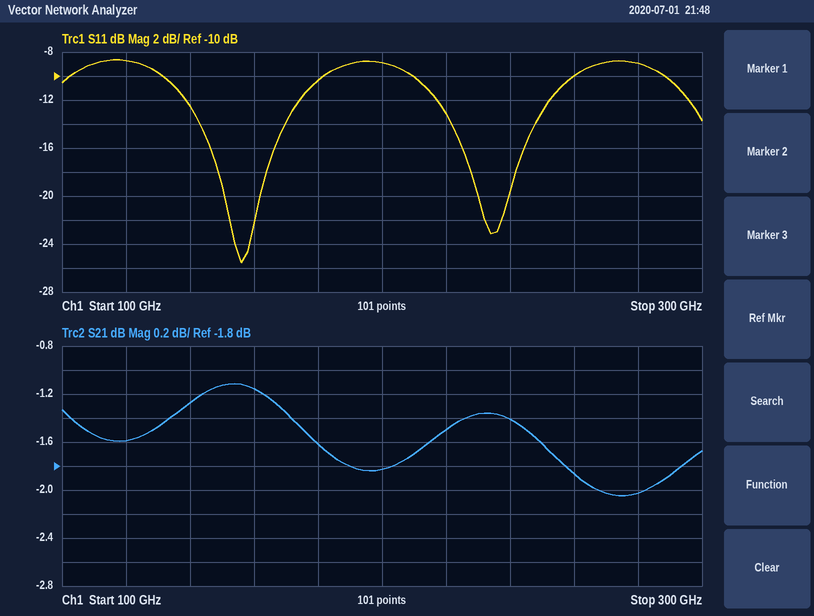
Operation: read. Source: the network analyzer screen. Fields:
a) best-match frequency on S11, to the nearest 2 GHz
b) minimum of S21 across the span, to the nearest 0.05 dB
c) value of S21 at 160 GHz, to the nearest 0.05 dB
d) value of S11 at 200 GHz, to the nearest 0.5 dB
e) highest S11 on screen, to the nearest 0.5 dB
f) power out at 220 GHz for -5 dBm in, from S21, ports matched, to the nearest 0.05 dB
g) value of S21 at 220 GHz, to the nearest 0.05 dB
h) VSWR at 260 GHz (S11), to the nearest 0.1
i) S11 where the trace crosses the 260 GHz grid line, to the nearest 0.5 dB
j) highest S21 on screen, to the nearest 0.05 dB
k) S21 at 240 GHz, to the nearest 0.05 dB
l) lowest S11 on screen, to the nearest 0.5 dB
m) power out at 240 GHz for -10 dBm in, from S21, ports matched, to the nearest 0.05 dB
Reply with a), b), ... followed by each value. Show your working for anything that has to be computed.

a) 156 GHz
b) -2.05 dB
c) -1.15 dB
d) -9.0 dB
e) -8.5 dB
f) -5 dBm + (-1.50 dB) = -6.50 dBm
g) -1.50 dB
h) |Γ| = 10^(-10/20) = 0.3162; VSWR = (1 + 0.3162)/(1 − 0.3162) ≈ 1.9
i) -10.0 dB
j) -1.10 dB
k) -1.40 dB
l) -25.5 dB
m) -10 dBm + (-1.40 dB) = -11.40 dBm
